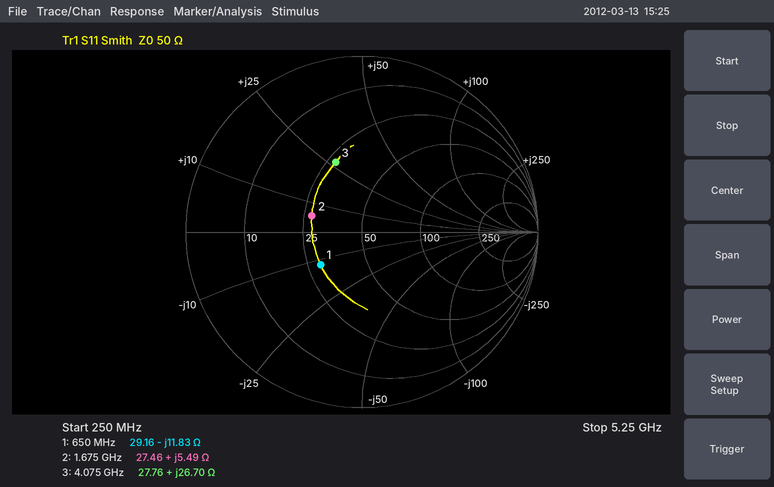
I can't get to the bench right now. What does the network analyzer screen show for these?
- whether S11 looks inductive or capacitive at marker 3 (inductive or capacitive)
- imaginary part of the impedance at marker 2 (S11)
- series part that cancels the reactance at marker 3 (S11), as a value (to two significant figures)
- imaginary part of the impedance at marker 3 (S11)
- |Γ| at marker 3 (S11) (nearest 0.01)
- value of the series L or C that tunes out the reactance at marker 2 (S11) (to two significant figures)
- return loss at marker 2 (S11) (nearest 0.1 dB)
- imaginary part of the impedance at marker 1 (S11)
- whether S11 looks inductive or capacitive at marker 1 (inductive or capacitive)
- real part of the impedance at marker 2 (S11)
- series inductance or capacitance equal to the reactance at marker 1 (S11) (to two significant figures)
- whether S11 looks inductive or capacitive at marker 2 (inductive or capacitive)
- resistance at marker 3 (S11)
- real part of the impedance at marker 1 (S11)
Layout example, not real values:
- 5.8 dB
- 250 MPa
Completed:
- inductive
- +5.49 Ω
- 1.5 pF
- +26.70 Ω
- 0.42
- 17 pF
- 10.5 dB
- -11.83 Ω
- capacitive
- 27.46 Ω
- 21 pF
- inductive
- 27.76 Ω
- 29.16 Ω
